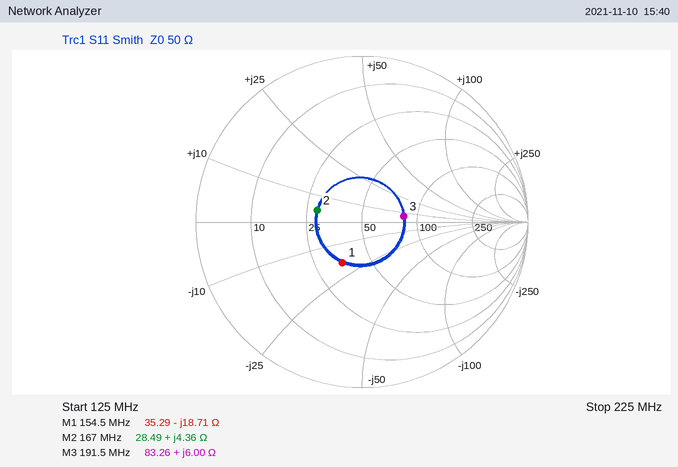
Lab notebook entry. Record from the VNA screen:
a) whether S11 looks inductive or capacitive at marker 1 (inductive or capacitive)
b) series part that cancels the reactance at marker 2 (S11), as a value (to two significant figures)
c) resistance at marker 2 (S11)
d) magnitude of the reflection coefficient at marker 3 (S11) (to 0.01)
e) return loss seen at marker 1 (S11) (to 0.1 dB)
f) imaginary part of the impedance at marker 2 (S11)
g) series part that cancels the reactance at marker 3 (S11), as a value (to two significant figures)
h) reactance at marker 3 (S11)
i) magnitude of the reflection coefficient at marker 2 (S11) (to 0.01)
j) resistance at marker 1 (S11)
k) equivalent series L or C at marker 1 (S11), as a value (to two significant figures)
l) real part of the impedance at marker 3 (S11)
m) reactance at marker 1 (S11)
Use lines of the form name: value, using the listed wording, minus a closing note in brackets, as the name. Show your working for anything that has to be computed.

whether S11 looks inductive or capacitive at marker 1: capacitive
series part that cancels the reactance at marker 2 (S11), as a value: C = 1/(2π × 167 MHz × 4.36 Ω) ≈ 219 pF, so 220 pF to two significant figures
resistance at marker 2: 28.49 Ω
magnitude of the reflection coefficient at marker 3 (S11): 0.25
return loss seen at marker 1 (S11): 11.3 dB
imaginary part of the impedance at marker 2: +4.36 Ω
series part that cancels the reactance at marker 3 (S11), as a value: C = 1/(2π × 191.5 MHz × 6 Ω) ≈ 139 pF, so 140 pF to two significant figures
reactance at marker 3: +6.00 Ω
magnitude of the reflection coefficient at marker 2 (S11): 0.28
resistance at marker 1: 35.29 Ω
equivalent series L or C at marker 1 (S11), as a value: C = 1/(2π × 154.5 MHz × 18.71 Ω) ≈ 55 pF
real part of the impedance at marker 3: 83.26 Ω
reactance at marker 1: -18.71 Ω
